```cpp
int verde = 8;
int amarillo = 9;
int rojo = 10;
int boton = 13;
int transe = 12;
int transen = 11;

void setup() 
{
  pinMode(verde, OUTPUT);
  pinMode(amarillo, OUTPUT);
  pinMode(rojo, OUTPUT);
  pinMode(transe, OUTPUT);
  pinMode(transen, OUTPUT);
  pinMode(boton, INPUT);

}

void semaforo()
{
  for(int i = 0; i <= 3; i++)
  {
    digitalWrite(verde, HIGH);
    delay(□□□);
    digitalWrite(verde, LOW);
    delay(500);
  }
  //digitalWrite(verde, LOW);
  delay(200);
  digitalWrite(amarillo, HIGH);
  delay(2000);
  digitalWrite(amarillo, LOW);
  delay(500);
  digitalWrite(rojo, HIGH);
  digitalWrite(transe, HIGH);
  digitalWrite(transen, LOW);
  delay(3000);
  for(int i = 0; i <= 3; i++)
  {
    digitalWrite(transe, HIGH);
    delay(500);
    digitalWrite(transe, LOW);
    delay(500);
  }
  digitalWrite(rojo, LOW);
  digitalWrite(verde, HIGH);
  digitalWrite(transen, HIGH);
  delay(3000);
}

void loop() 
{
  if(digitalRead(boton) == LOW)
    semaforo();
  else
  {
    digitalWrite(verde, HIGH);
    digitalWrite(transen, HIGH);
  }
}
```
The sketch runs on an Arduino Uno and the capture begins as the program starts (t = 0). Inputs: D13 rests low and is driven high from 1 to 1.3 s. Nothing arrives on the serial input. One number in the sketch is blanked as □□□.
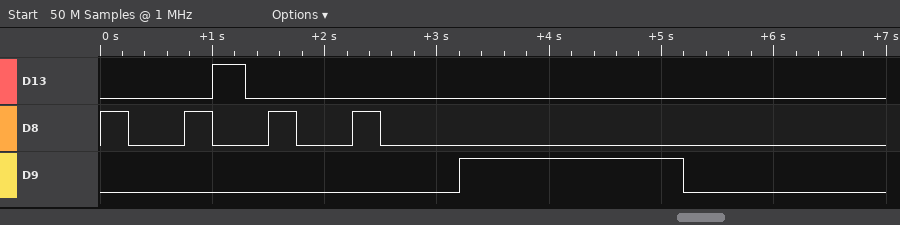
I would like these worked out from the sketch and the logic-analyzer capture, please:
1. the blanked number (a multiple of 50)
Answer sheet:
250
